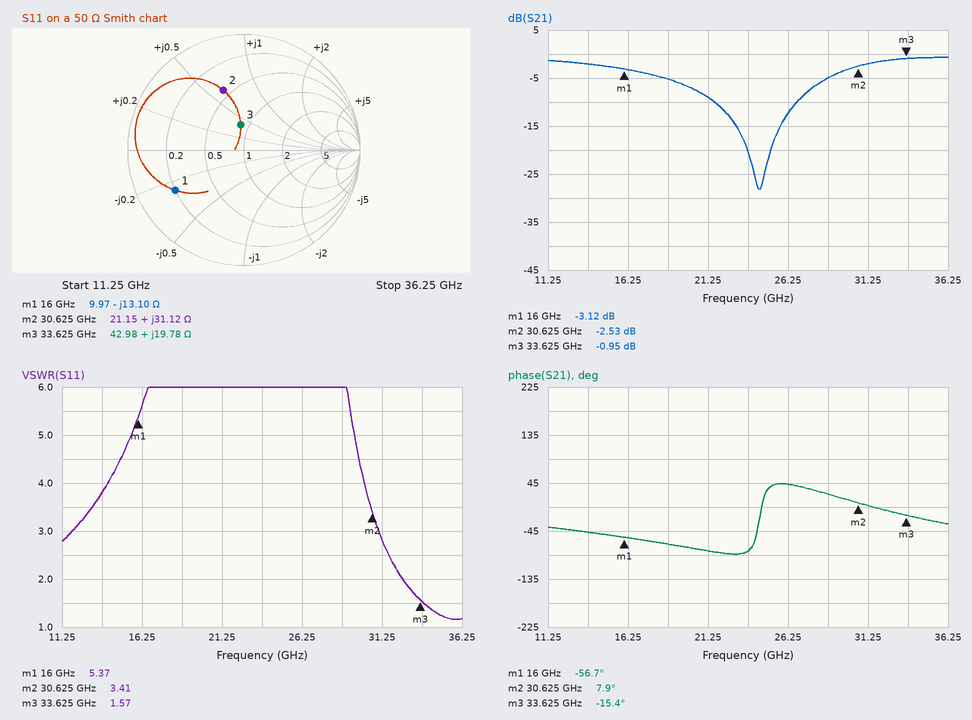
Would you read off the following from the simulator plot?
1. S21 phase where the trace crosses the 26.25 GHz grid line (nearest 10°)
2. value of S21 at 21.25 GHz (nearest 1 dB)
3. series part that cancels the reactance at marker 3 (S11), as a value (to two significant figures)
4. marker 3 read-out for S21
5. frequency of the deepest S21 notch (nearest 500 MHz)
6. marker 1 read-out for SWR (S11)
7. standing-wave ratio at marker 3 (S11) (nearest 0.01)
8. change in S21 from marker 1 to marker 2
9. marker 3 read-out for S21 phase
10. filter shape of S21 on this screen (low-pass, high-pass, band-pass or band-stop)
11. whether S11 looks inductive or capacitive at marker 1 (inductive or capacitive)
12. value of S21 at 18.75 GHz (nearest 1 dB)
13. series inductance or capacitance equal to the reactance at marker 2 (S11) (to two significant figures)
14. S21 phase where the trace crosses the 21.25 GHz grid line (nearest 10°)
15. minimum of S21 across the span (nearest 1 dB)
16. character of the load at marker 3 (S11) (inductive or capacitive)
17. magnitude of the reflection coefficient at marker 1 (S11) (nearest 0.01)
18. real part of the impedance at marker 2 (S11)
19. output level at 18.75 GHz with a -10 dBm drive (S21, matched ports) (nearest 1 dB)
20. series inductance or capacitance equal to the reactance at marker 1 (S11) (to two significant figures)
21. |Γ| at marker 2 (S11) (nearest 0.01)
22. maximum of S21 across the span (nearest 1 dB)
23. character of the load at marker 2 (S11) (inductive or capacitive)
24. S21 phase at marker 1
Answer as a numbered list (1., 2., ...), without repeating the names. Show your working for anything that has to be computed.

1. 40°
2. -9 dB
3. C = 1/(2π × 33.625 GHz × 19.78 Ω) ≈ 239 fF, so 240 fF to two significant figures
4. -0.95 dB
5. 24.5 GHz
6. 5.37
7. 1.57
8. -2.53 − (-3.12) = 0.59 dB
9. -15.4°
10. band-stop
11. capacitive
12. -5 dB
13. L = 31.12 Ω/(2π × 30.625 GHz) ≈ 162 pH, so 160 pH to two significant figures
14. -80°
15. -28 dB
16. inductive
17. 0.69
18. 21.15 Ω
19. -10 dBm + (-5 dB) = -15 dBm
20. C = 1/(2π × 16 GHz × 13.1 Ω) ≈ 759 fF, so 760 fF to two significant figures
21. 0.55
22. -1 dB
23. inductive
24. -56.7°
